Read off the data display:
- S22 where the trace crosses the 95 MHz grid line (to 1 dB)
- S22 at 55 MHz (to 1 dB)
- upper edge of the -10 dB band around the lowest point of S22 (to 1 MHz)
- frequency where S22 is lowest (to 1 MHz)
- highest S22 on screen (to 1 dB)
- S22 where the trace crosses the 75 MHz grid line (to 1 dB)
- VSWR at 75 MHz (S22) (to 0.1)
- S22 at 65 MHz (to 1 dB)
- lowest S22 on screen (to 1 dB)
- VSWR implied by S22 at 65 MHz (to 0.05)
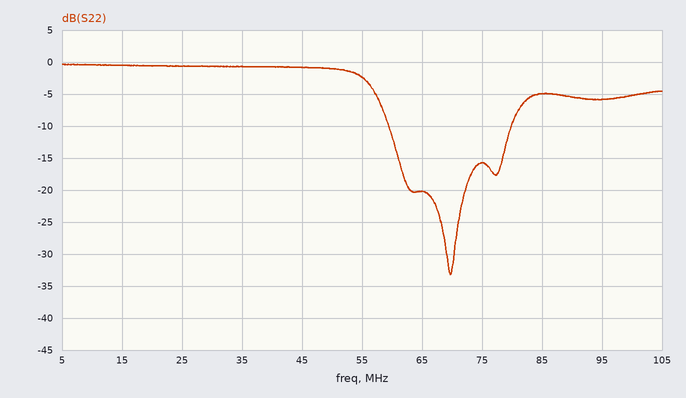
-6 dB
-2 dB
80 MHz
70 MHz
0 dB
-16 dB
1.4
-20 dB
-33 dB
1.20
